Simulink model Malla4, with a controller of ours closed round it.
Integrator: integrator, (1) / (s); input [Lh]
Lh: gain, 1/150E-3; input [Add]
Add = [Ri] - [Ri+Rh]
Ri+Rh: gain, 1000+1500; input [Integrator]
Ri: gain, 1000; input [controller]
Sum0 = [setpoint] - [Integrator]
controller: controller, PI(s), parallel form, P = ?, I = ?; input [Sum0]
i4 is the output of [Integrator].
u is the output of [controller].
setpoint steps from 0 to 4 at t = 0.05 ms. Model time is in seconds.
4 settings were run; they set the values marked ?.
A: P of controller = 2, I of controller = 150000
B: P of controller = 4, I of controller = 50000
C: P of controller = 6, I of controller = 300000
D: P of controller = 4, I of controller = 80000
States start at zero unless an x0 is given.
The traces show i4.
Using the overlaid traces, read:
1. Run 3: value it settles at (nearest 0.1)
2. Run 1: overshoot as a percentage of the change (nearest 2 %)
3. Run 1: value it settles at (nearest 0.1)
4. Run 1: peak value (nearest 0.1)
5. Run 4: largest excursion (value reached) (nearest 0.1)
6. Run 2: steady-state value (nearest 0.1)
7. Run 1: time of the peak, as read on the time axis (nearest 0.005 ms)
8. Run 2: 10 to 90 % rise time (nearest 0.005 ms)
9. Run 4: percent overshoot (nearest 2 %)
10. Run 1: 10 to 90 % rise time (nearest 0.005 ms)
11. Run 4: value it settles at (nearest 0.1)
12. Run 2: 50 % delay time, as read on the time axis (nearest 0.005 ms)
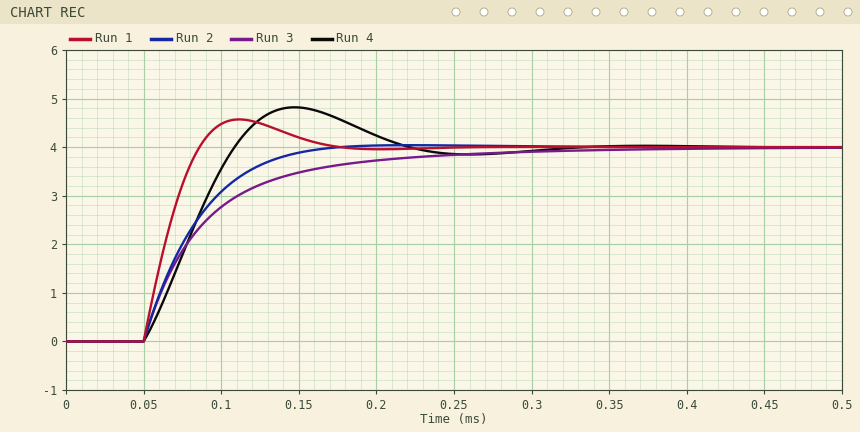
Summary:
4.0
14 %
4.0
4.6
4.8
4.0
0.110 ms
0.070 ms
20 %
0.025 ms
4.0
0.075 ms
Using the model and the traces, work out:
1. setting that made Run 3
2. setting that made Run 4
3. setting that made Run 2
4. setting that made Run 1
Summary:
B
A
D
C
